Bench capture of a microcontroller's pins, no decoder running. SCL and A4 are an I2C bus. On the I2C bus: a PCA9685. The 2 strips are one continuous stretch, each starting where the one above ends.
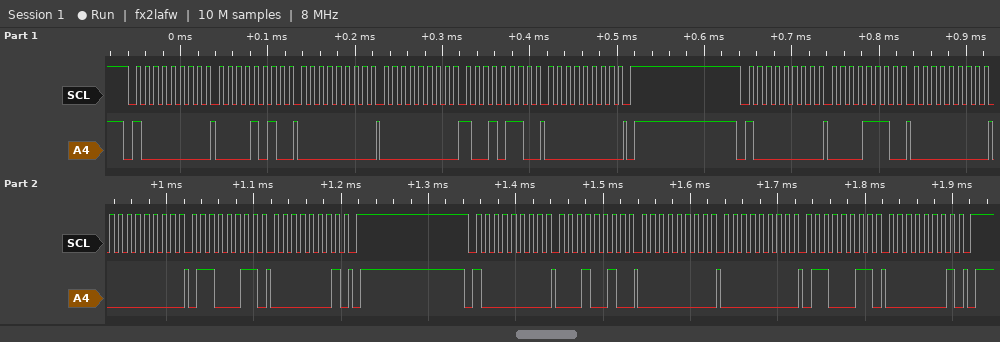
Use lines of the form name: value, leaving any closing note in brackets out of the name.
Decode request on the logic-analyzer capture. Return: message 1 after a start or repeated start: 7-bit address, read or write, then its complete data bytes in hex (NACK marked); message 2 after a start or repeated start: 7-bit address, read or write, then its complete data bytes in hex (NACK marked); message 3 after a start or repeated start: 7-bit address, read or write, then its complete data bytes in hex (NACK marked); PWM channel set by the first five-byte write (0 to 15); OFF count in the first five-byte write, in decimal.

message 1 after a start or repeated start: 7-bit address, read or write, then its complete data bytes in hex: 0x40 write: 0A 00 00 96 00
message 2 after a start or repeated start: 7-bit address, read or write, then its complete data bytes in hex: 0x40 write: 0E 00 00 63 01
message 3 after a start or repeated start: 7-bit address, read or write, then its complete data bytes in hex: 0x40 write: 12 00 00 63 01
PWM channel set by the first five-byte write: 1
OFF count in the first five-byte write, in decimal: 150
